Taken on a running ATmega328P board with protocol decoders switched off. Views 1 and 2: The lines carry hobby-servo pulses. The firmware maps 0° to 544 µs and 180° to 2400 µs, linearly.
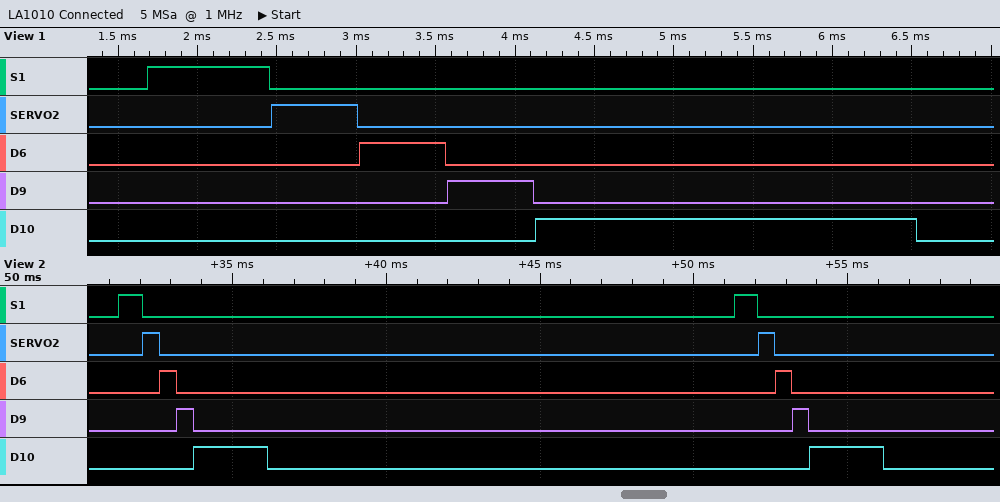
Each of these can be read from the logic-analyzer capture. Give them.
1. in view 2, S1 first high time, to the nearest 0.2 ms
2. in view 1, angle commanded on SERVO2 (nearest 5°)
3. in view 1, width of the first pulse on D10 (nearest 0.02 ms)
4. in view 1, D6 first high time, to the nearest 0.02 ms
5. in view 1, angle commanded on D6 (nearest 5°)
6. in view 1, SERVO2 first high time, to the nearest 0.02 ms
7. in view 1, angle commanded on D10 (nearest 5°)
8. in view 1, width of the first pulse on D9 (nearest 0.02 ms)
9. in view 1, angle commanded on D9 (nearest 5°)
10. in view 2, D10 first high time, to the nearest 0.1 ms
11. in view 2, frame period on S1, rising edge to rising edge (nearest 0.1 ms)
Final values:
0.8 ms
0°
2.40 ms
0.54 ms
0°
0.54 ms
180°
0.54 ms
0°
2.4 ms
20.0 ms
